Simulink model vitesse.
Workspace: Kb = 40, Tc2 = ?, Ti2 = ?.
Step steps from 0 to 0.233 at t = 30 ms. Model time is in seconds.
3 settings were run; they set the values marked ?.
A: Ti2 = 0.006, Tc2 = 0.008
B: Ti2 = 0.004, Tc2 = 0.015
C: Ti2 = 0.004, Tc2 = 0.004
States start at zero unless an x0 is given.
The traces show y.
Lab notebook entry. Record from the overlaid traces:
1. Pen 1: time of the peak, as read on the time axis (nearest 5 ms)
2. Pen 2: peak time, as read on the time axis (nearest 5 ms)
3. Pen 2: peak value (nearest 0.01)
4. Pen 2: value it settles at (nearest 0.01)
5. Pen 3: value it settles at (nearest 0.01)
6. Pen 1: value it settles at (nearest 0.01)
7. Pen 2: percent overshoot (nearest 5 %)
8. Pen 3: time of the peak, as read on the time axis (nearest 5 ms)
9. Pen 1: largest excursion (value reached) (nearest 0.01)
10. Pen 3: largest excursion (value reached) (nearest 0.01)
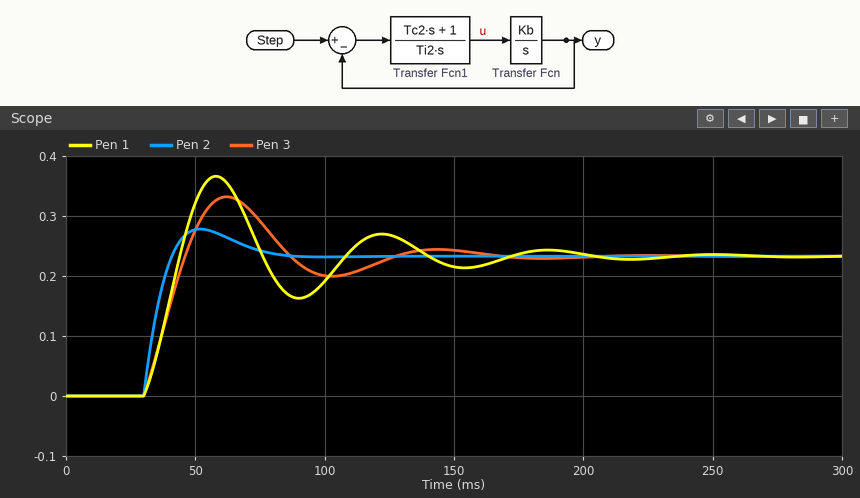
60 ms
50 ms
0.28
0.23
0.23
0.23
20 %
60 ms
0.37
0.33
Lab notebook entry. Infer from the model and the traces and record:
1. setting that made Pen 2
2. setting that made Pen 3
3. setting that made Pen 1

B
A
C
